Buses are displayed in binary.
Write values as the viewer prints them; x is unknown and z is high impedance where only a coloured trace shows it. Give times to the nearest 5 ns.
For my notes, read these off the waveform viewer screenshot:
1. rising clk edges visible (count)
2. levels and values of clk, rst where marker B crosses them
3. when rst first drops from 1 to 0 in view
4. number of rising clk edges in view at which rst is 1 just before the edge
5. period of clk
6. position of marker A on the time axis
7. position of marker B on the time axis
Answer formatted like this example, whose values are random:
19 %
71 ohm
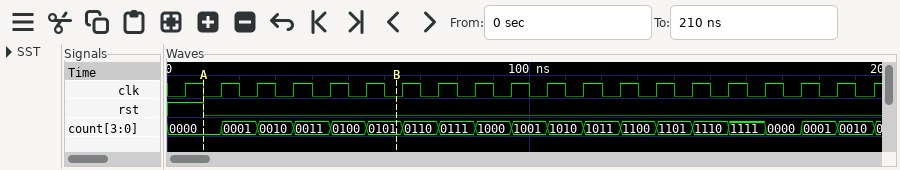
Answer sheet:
20
clk=0, rst=0
10 ns
1
10 ns
10 ns
65 ns
